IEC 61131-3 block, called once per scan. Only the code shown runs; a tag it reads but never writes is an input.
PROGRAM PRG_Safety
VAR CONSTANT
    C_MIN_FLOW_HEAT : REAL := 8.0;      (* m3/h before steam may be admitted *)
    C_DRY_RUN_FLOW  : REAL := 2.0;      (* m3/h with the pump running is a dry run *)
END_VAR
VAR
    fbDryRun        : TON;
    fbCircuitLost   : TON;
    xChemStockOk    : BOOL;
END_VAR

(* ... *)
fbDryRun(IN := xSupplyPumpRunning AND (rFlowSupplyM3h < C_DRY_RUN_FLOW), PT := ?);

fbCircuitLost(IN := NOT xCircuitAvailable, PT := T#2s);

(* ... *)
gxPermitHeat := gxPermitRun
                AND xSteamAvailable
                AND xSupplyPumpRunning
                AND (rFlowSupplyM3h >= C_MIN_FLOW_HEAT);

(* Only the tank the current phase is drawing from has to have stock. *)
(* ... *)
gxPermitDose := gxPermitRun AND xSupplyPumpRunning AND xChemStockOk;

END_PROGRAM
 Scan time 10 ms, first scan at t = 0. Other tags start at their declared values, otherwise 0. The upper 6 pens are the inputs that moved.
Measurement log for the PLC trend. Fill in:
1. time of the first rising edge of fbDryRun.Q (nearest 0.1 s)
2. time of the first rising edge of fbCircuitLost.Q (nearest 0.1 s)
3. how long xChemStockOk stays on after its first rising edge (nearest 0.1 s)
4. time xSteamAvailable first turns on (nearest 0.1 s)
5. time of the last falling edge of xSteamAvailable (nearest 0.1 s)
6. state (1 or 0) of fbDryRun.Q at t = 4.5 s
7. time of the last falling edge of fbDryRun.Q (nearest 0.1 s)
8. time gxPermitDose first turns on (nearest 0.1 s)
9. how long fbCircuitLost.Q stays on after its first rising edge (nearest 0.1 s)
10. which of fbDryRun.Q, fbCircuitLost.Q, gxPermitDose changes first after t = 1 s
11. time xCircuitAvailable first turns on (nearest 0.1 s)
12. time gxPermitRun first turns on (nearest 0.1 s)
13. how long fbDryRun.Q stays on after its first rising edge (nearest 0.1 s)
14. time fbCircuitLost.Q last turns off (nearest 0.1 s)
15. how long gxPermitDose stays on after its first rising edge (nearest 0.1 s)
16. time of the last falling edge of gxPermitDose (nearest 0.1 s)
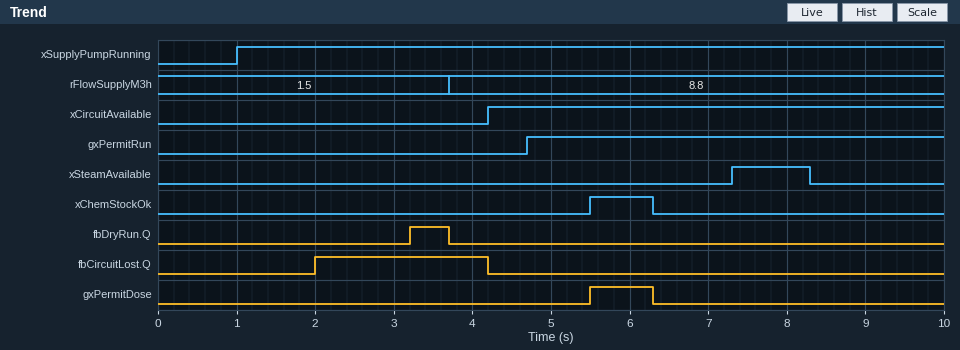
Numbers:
3.2 s
2.0 s
0.8 s
7.3 s
8.3 s
0
3.7 s
5.5 s
2.2 s
fbCircuitLost.Q
4.2 s
4.7 s
0.5 s
4.2 s
0.8 s
6.3 s
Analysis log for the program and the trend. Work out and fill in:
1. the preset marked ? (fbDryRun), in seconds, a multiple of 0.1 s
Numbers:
2.2 s
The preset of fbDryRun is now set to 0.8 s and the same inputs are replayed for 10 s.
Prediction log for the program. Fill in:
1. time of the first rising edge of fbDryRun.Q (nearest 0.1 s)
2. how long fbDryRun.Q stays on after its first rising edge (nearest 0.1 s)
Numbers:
1.8 s
1.9 s
